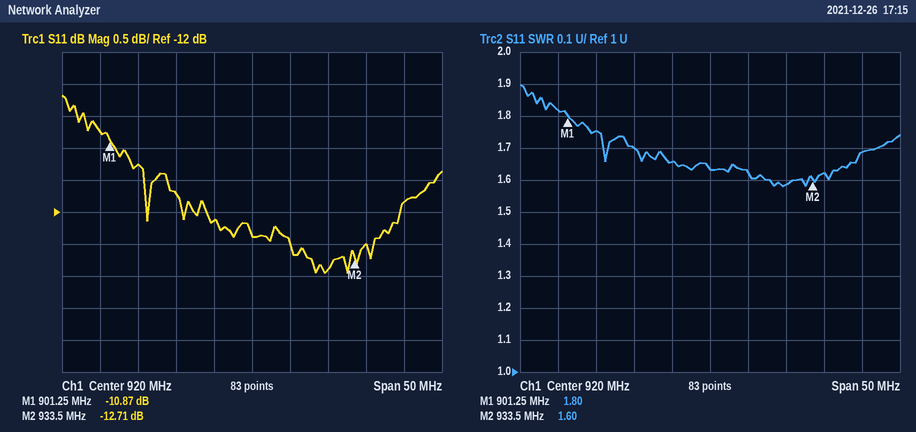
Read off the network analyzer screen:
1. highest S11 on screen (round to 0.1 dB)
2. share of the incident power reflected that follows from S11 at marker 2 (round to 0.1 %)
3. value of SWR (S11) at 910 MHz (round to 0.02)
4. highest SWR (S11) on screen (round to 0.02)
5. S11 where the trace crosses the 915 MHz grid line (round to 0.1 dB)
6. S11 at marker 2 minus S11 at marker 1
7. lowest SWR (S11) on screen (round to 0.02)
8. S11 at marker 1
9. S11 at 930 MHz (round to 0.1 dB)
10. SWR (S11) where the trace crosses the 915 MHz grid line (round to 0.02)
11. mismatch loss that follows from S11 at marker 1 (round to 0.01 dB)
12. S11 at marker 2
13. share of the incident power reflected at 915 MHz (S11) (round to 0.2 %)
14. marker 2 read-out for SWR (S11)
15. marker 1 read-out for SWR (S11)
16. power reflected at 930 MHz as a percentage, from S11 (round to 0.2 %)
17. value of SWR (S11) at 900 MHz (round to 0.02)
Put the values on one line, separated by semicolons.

-10.2 dB; 5.4 %; 1.70; 1.90; -12.1 dB; -1.84 dB; 1.58; -10.87 dB; -12.9 dB; 1.66; 0.37 dB; -12.71 dB; 6.2 %; 1.60; 1.80; 5.2 %; 1.82
